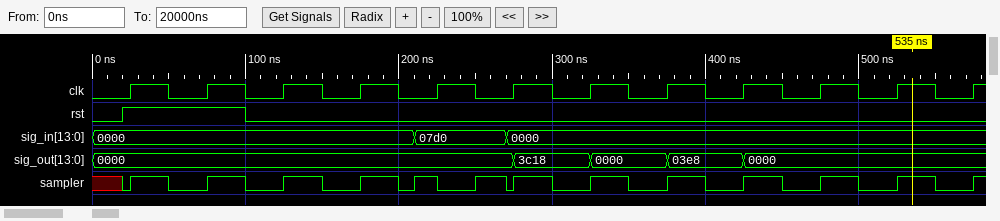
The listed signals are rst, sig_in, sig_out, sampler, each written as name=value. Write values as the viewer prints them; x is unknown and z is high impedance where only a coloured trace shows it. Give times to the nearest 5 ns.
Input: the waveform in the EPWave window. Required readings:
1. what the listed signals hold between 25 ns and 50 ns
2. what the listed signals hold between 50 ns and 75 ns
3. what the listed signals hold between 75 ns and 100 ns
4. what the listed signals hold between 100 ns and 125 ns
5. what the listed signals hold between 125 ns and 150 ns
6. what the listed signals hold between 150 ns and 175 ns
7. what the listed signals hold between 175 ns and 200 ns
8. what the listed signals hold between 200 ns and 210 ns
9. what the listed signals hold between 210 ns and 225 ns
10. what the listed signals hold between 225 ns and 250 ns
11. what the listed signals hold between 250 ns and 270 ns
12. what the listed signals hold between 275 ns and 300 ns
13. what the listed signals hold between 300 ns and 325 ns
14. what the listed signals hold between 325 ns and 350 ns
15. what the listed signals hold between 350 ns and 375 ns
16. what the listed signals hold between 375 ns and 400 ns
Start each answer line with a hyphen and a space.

- rst=1, sig_in=0000, sig_out=0000, sampler=1
- rst=1, sig_in=0000, sig_out=0000, sampler=0
- rst=1, sig_in=0000, sig_out=0000, sampler=1
- rst=0, sig_in=0000, sig_out=0000, sampler=0
- rst=0, sig_in=0000, sig_out=0000, sampler=1
- rst=0, sig_in=0000, sig_out=0000, sampler=0
- rst=0, sig_in=0000, sig_out=0000, sampler=1
- rst=0, sig_in=0000, sig_out=0000, sampler=0
- rst=0, sig_in=07d0, sig_out=0000, sampler=1
- rst=0, sig_in=07d0, sig_out=0000, sampler=0
- rst=0, sig_in=07d0, sig_out=0000, sampler=1
- rst=0, sig_in=0000, sig_out=3c18, sampler=1
- rst=0, sig_in=0000, sig_out=3c18, sampler=0
- rst=0, sig_in=0000, sig_out=0000, sampler=1
- rst=0, sig_in=0000, sig_out=0000, sampler=0
- rst=0, sig_in=0000, sig_out=03e8, sampler=1
